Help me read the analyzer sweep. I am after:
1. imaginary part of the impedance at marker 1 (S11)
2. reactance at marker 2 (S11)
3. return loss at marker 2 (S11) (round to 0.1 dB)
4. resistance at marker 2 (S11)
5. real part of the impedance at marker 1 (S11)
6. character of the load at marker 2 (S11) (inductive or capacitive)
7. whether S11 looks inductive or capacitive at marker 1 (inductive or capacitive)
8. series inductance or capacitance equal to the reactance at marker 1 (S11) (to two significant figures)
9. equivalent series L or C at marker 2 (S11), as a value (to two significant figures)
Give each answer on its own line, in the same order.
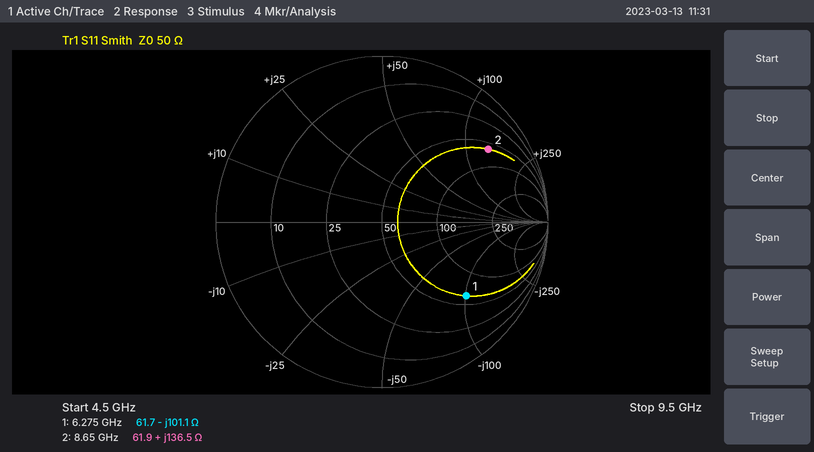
-101.1 Ω
+136.5 Ω
2.2 dB
61.9 Ω
61.7 Ω
inductive
capacitive
250 fF
2.5 nH
